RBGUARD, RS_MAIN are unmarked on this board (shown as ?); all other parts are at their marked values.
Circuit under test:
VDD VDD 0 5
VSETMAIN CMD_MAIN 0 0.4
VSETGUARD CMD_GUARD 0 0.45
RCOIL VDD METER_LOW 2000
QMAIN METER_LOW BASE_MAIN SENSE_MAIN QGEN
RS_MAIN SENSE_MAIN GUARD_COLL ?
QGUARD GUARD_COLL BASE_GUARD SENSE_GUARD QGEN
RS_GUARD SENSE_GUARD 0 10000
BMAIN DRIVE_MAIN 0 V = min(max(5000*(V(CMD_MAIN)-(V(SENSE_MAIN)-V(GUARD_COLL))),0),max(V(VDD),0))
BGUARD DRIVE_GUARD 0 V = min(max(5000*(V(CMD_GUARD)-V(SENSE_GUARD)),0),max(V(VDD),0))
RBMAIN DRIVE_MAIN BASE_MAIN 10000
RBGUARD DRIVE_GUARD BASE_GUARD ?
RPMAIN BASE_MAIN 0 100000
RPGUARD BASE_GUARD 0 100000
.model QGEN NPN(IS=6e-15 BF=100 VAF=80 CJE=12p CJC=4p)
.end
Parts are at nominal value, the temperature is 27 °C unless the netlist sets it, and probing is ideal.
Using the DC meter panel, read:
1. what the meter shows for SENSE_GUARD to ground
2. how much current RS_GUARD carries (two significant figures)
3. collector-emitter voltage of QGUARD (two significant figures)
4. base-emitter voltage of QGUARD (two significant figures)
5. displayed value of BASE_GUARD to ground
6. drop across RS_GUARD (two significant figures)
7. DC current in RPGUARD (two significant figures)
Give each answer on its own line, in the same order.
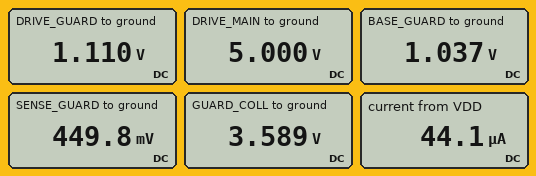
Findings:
449.8 mV
45 µA
3.1 V
590 mV
1.037 V
450 mV
10 µA
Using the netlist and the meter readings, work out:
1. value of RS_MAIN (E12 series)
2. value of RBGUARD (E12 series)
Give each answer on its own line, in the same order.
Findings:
8.2 kΩ
6.8 kΩ
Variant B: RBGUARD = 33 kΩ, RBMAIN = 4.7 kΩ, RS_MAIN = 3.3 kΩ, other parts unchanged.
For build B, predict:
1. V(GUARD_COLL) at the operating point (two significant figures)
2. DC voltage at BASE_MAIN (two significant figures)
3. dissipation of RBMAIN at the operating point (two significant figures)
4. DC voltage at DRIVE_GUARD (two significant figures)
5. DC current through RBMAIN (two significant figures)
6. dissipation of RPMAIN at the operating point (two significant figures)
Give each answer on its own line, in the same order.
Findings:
4.0 V
4.8 V
11 µW
1.4 V
48 µA
230 µW
